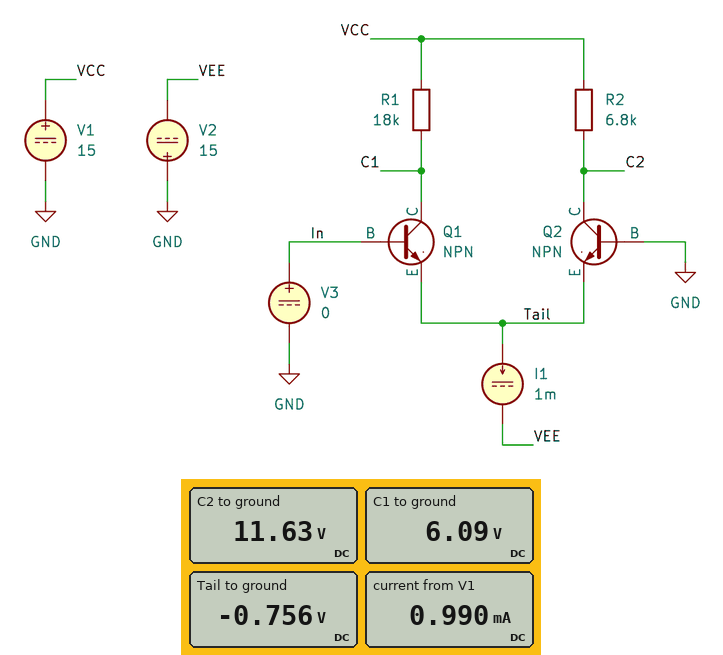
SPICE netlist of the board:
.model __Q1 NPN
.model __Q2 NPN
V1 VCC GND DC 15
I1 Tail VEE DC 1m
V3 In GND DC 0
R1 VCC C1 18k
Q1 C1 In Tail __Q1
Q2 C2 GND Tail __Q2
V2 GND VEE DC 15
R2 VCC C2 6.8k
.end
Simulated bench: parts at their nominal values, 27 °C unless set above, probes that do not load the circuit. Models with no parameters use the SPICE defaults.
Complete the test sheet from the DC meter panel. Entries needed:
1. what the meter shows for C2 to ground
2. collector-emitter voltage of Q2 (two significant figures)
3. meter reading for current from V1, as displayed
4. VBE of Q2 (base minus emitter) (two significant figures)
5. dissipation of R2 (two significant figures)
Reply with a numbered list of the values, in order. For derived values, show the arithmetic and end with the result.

1. 11.63 V
2. 11.63 V - (-756 mV) = 12 V
3. 0.990 mA
4. 0 V - (-756 mV) = 760 mV
5. (15 V - 11.63 V)^2 / 6.8 kΩ = 1.7 mW
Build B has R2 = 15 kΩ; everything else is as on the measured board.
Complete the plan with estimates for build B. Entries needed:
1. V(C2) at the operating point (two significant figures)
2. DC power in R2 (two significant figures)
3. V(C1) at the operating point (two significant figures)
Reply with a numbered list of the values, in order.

1. 7.6 V
2. 3.7 mW
3. 6.1 V
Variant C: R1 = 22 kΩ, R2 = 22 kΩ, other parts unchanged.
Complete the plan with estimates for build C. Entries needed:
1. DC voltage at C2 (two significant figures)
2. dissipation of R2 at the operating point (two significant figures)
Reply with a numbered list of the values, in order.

1. 4.1 V
2. 5.4 mW
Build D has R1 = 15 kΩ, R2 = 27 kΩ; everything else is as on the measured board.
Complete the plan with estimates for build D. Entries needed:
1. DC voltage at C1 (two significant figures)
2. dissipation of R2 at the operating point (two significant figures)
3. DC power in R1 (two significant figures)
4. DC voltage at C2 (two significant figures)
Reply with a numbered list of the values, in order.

1. 7.6 V
2. 6.6 mW
3. 3.7 mW
4. 1.6 V
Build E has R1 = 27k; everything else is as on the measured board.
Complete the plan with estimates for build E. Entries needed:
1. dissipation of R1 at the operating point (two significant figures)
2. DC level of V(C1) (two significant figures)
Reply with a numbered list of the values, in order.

1. 6.6 mW
2. 1.6 V
